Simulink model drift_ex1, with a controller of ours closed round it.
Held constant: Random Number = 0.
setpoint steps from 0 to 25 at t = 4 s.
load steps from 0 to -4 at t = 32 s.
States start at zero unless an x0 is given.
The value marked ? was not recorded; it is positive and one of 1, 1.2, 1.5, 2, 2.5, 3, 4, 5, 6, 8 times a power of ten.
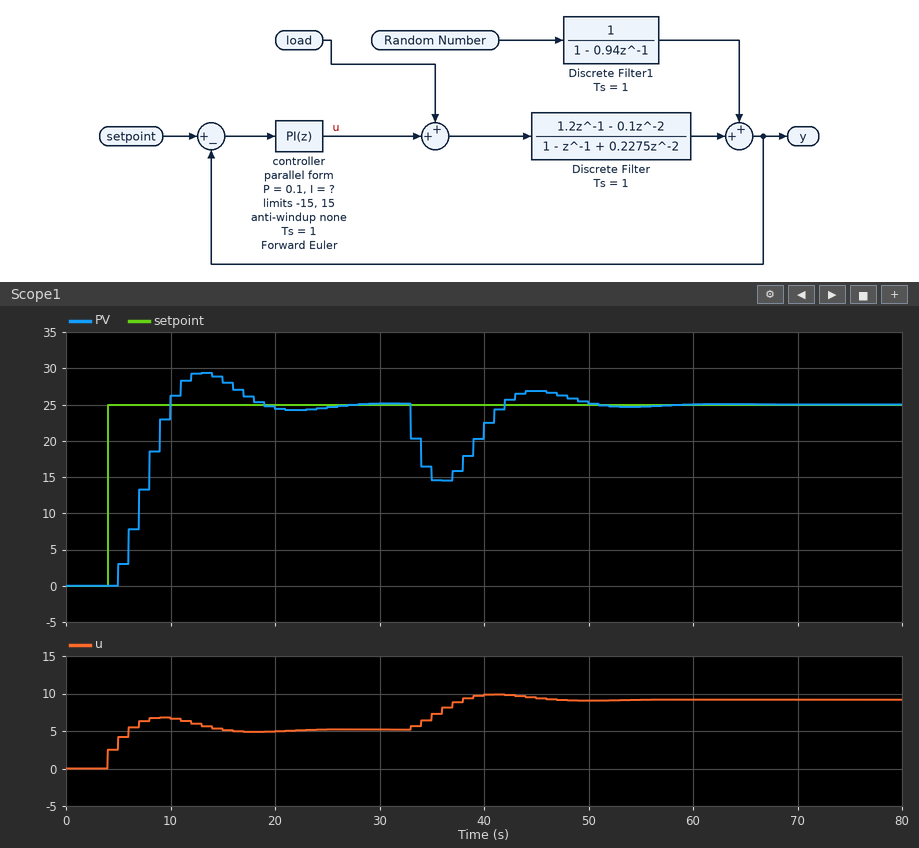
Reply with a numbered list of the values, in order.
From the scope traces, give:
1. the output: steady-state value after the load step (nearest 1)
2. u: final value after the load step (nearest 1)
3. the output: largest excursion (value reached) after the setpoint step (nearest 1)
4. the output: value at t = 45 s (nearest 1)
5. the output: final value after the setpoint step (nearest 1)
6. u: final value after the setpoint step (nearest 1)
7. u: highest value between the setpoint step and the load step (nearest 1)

1. 25
2. 9
3. 29
4. 27
5. 25
6. 5
7. 7
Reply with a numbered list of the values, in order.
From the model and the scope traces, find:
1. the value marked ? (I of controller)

1. 0.08
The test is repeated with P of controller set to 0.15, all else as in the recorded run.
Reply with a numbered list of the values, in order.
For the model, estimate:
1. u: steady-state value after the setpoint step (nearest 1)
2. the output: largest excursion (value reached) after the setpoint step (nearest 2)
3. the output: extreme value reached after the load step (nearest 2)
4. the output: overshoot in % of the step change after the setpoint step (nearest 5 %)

1. 5
2. 28
3. 16
4. 10 %
